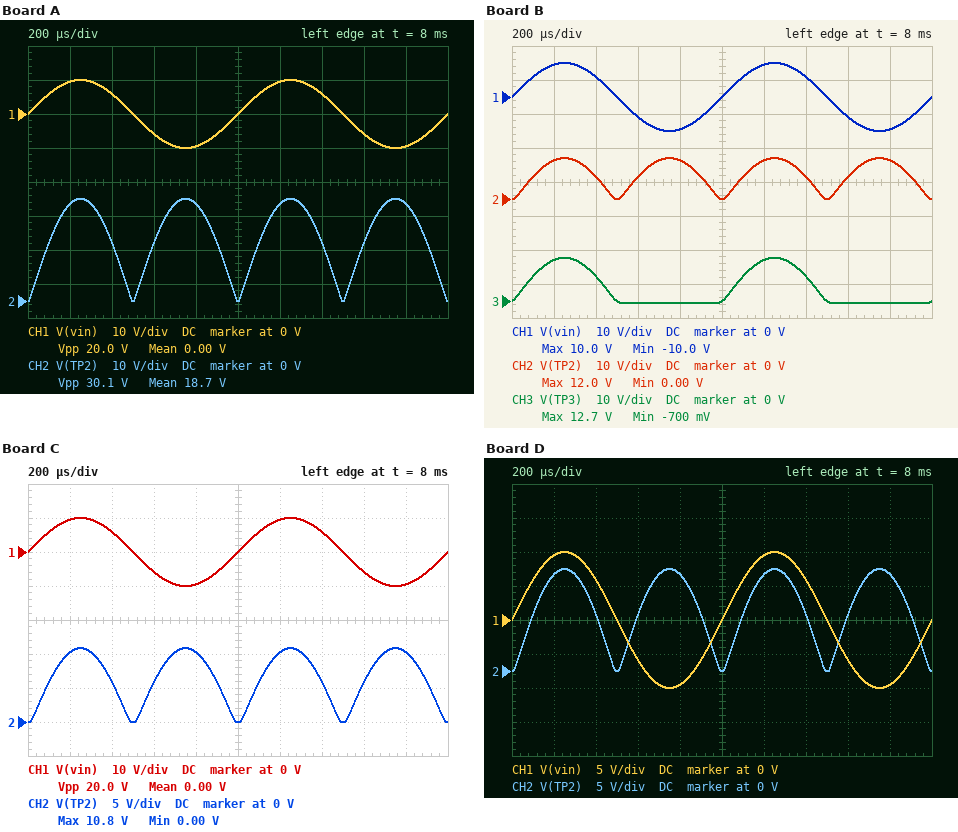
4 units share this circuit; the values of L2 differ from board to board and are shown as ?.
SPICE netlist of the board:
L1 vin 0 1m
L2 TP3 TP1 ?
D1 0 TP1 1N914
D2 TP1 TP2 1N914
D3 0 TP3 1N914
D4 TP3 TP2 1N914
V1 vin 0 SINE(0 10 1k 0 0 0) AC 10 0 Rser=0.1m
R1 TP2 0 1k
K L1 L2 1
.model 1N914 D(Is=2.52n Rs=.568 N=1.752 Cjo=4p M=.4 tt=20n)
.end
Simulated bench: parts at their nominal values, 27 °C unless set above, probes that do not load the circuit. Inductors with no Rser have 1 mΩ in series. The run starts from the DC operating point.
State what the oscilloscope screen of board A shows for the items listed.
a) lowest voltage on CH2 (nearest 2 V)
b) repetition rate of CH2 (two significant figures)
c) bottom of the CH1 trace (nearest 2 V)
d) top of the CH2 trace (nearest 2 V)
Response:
0 V
2.0 kHz
-10 V
30 V
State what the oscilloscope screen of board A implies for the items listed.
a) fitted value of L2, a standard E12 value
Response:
10 mH
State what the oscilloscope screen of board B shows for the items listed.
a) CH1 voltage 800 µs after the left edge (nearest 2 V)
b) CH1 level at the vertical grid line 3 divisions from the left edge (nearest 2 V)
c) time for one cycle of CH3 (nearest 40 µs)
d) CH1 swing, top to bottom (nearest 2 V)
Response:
-10 V
-6 V
1.00 ms
20 V
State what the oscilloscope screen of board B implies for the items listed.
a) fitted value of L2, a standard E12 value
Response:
1.8 mH
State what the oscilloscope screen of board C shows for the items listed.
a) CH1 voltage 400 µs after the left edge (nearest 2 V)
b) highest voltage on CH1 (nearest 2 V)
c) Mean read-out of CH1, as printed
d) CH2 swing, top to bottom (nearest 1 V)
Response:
6 V
10 V
0.00 V
11 V
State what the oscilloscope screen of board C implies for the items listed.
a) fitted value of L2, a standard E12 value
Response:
1.5 mH
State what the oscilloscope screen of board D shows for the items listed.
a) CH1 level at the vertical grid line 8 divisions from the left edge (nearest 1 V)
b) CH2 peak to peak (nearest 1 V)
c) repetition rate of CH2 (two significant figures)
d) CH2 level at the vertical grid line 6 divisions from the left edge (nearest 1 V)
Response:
-6 V
15 V
2.0 kHz
14 V
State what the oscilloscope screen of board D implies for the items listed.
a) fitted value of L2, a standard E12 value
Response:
2.7 mH
